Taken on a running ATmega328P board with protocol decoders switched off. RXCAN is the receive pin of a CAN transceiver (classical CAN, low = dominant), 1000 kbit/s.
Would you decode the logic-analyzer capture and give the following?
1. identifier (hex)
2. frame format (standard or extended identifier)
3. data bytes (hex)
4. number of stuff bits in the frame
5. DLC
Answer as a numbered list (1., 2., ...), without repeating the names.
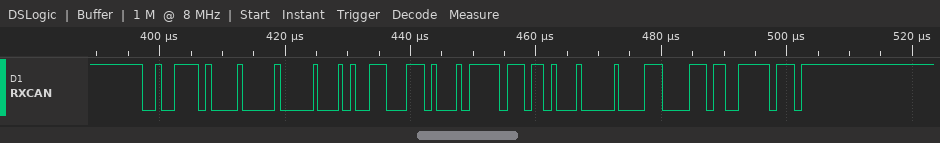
1. 0x27A
2. standard
3. 00 29 C7 45 FE D1 00 70
4. 5
5. 8
